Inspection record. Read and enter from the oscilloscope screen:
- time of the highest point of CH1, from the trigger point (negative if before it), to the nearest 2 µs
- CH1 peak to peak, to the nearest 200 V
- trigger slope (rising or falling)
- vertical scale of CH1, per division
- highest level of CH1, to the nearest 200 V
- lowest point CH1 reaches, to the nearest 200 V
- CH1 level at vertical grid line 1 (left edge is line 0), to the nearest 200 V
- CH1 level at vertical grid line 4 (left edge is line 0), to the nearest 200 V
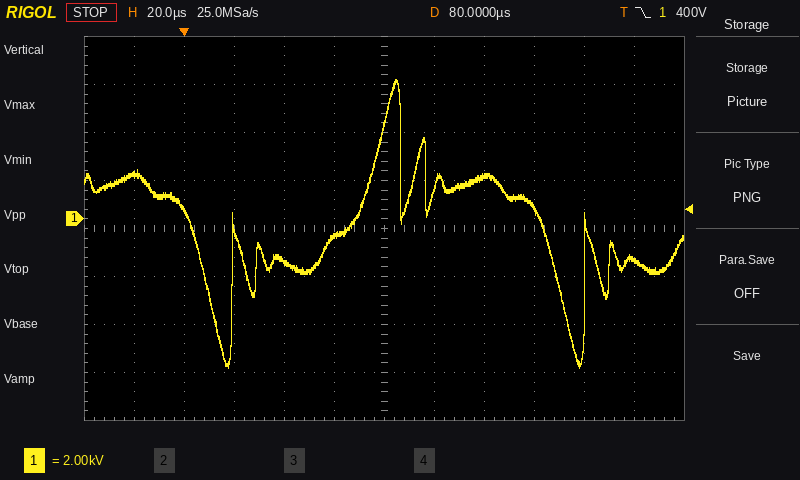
+84 µs
12.0 kV
falling
2 kV
5.8 kV
-6.2 kV
1.8 kV
-1.8 kV
